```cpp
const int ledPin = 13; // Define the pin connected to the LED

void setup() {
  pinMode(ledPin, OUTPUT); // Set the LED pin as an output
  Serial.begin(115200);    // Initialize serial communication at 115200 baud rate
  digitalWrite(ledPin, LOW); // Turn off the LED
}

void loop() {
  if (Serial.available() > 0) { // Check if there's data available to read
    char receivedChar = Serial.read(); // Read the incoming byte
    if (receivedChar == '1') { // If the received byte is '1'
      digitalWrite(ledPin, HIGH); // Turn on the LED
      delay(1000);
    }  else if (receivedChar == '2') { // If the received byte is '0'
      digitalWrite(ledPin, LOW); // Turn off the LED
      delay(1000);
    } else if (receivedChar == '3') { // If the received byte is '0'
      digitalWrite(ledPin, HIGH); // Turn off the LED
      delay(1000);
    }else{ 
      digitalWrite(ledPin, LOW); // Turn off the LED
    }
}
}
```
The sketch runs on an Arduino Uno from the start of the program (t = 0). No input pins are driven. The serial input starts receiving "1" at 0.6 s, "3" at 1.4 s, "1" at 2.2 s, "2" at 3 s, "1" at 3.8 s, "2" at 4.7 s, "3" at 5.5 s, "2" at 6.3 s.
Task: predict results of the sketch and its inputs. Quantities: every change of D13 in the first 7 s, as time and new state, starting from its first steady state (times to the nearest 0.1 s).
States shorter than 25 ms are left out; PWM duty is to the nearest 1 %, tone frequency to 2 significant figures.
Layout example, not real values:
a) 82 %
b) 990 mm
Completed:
a) 0 s low; 0.6 s high; 3.6 s low; 4.6 s high; 5.6 s low; 6.6 s high
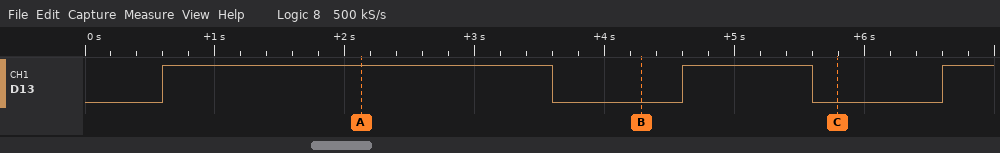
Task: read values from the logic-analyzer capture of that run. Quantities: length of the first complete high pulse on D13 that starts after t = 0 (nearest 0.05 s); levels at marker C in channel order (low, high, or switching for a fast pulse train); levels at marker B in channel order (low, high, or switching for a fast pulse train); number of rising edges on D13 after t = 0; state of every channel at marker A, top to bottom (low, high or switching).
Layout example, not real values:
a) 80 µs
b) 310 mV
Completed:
a) 3.00 s
b) D13 low
c) D13 low
d) 3
e) D13 high
